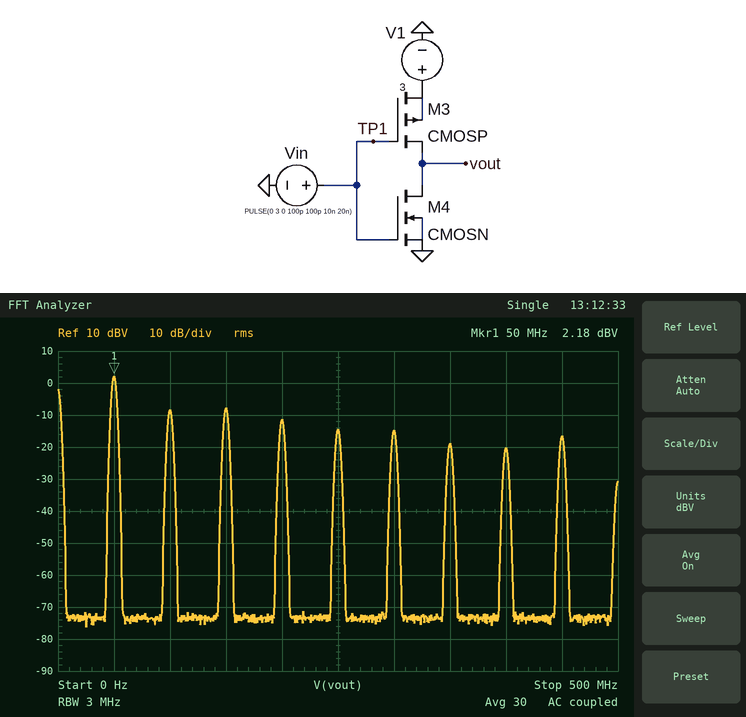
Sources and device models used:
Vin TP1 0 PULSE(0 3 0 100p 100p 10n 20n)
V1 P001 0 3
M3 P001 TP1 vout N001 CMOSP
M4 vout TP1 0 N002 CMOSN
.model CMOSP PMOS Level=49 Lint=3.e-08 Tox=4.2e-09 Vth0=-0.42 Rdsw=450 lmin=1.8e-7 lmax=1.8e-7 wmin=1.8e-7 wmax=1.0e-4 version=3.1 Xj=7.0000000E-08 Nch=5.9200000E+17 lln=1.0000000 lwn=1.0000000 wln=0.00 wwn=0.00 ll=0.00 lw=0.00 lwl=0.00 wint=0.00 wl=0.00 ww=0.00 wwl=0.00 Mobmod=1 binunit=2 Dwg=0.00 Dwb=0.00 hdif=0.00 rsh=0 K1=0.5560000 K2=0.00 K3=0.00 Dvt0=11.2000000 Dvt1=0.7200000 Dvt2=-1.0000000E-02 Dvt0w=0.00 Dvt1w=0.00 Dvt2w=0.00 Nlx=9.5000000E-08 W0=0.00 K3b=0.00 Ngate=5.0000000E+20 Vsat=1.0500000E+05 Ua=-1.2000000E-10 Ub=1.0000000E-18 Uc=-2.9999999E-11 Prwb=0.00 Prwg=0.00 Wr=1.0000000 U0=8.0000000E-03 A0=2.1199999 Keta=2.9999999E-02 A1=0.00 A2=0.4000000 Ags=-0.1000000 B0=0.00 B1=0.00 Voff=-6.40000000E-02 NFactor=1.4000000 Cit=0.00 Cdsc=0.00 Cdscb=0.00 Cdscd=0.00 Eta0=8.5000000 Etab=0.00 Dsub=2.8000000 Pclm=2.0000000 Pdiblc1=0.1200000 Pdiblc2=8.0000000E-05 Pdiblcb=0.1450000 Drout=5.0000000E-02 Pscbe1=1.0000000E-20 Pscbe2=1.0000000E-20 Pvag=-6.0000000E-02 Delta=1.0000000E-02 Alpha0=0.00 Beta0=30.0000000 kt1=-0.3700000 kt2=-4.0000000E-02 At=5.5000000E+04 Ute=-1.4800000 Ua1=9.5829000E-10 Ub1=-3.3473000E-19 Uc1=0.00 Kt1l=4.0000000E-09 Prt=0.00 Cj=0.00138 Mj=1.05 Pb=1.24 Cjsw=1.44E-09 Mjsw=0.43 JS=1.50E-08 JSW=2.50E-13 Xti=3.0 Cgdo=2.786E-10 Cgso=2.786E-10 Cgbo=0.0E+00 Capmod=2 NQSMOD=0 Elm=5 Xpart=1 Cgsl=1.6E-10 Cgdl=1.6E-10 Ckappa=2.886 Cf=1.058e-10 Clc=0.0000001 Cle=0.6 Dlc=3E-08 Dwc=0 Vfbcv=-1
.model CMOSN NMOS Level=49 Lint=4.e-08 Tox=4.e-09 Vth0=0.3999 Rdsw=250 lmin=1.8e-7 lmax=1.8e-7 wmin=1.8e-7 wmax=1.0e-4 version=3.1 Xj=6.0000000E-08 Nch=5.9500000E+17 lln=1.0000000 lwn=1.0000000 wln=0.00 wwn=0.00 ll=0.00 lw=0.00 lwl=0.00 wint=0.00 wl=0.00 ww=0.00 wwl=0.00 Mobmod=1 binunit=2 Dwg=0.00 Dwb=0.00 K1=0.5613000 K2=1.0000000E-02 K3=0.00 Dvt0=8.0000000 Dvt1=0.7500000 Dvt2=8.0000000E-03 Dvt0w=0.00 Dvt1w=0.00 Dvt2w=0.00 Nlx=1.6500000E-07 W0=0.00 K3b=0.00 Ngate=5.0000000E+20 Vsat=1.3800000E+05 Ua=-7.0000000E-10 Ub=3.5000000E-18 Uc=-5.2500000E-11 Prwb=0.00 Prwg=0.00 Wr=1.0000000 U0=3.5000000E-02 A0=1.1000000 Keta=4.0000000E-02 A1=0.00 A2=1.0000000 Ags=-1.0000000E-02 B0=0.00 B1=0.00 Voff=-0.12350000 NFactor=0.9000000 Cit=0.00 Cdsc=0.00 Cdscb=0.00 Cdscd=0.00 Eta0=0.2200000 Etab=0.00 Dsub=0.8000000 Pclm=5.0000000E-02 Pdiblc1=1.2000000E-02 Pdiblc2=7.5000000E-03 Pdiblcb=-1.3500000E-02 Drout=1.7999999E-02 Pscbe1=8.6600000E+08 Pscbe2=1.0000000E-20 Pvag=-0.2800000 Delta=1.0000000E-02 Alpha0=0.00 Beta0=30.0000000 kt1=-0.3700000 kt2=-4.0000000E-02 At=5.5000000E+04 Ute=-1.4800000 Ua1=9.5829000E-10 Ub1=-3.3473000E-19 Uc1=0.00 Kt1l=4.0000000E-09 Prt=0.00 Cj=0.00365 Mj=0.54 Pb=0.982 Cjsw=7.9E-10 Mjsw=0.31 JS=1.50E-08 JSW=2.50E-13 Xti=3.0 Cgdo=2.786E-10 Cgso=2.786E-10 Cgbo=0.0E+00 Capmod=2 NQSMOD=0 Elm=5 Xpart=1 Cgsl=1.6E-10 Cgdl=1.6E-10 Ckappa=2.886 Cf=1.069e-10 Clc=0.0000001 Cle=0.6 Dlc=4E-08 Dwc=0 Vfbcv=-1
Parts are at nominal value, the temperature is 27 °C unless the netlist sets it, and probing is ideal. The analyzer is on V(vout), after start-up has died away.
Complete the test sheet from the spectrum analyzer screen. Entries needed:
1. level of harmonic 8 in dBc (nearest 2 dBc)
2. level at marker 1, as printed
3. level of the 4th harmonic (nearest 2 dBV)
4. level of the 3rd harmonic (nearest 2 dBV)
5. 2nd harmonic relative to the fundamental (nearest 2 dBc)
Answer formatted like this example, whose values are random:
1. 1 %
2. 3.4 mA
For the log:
1. -22 dBc
2. 2.18 dBV
3. -12 dBV
4. -8 dBV
5. -10 dBc
